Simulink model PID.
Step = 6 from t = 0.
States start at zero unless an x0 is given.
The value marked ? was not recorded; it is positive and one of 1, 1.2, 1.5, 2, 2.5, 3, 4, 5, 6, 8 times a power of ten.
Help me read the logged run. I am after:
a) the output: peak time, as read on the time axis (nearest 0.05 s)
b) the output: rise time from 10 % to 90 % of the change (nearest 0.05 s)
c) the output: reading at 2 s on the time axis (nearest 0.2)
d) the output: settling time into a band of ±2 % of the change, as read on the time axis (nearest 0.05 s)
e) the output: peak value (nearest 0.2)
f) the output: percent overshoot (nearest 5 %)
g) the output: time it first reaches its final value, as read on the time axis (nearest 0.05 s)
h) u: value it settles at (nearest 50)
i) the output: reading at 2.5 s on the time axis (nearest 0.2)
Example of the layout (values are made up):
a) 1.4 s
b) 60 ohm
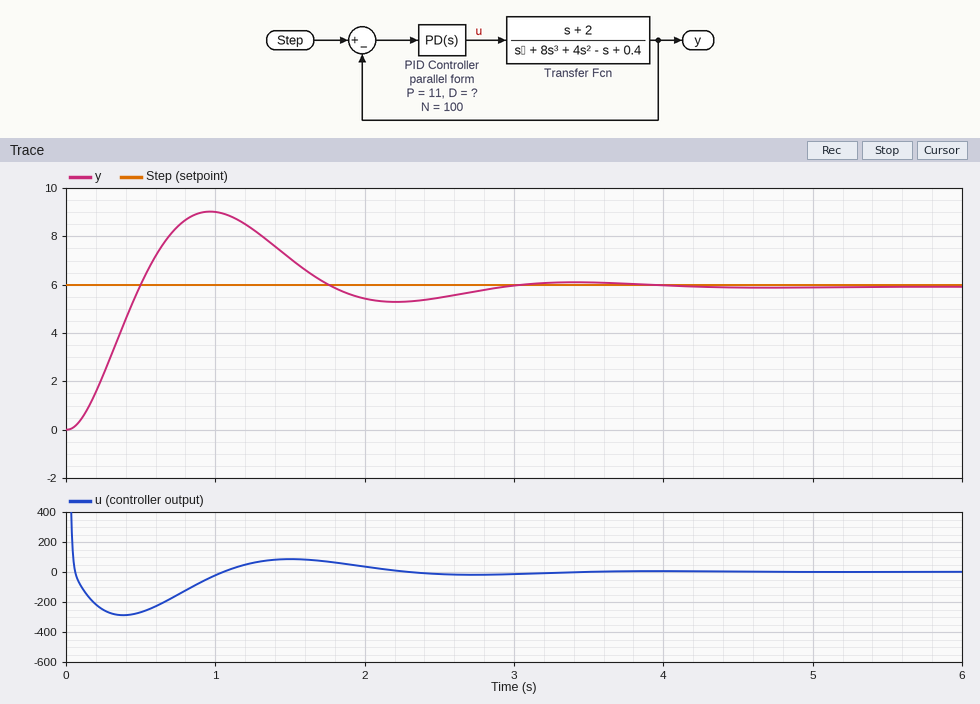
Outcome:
a) 0.95 s
b) 0.35 s
c) 5.4
d) 3.85 s
e) 9.0
f) 55 %
g) 0.50 s
h) 0
i) 5.4
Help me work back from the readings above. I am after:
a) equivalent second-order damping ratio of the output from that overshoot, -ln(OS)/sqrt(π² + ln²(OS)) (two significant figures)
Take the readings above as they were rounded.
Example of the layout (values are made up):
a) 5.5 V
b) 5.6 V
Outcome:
a) 0.19
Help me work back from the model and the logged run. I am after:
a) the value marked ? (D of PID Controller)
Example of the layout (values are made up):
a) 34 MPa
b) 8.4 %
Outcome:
a) 20
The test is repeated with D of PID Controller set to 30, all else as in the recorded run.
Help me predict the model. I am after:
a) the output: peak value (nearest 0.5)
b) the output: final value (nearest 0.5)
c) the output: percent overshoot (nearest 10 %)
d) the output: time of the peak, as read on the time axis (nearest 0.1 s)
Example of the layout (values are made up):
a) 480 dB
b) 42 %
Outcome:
a) 8.5
b) 6.0
c) 50 %
d) 0.7 s
